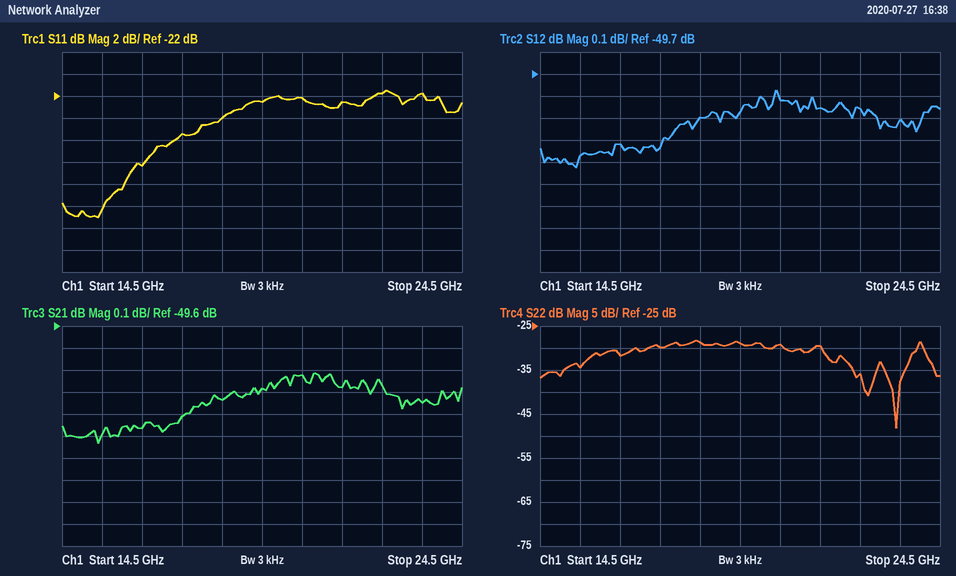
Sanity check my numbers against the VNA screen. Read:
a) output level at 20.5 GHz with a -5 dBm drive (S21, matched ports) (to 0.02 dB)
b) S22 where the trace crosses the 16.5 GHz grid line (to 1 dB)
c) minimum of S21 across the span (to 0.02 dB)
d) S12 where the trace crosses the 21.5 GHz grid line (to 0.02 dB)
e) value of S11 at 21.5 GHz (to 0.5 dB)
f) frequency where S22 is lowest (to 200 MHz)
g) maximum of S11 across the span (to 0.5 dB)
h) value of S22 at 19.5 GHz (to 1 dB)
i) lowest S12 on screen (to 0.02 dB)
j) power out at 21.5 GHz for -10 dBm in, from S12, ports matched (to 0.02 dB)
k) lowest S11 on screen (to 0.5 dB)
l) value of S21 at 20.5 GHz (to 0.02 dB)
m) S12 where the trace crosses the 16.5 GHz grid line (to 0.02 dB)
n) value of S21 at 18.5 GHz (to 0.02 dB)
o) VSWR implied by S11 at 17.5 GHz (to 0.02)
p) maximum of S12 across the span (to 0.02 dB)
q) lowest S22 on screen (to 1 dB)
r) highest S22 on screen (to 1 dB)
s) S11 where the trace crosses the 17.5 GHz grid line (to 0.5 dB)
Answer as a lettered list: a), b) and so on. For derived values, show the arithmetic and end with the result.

a) -5 dBm + (-49.82 dB) = -54.82 dBm
b) -32 dB
c) -50.14 dB
d) -49.86 dB
e) -22.5 dB
f) 23.4 GHz
g) -21.5 dB
h) -29 dB
i) -50.12 dB
j) -10 dBm + (-49.86 dB) = -59.86 dBm
k) -33.0 dB
l) -49.82 dB
m) -50.02 dB
n) -49.94 dB
o) |Γ| = 10^(-25.5/20) = 0.0531; VSWR = (1 + 0.0531)/(1 − 0.0531) ≈ 1.11, so 1.12 to the nearest 0.02
p) -49.78 dB
q) -48 dB
r) -28 dB
s) -25.5 dB
